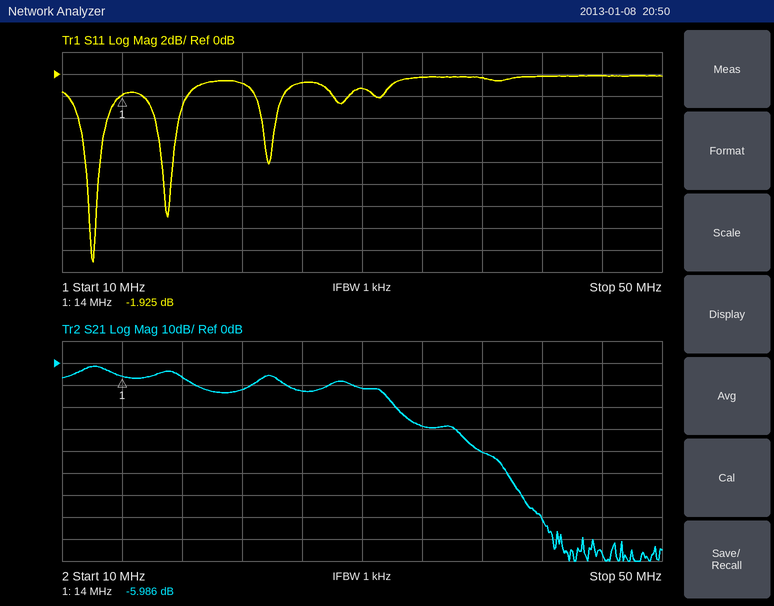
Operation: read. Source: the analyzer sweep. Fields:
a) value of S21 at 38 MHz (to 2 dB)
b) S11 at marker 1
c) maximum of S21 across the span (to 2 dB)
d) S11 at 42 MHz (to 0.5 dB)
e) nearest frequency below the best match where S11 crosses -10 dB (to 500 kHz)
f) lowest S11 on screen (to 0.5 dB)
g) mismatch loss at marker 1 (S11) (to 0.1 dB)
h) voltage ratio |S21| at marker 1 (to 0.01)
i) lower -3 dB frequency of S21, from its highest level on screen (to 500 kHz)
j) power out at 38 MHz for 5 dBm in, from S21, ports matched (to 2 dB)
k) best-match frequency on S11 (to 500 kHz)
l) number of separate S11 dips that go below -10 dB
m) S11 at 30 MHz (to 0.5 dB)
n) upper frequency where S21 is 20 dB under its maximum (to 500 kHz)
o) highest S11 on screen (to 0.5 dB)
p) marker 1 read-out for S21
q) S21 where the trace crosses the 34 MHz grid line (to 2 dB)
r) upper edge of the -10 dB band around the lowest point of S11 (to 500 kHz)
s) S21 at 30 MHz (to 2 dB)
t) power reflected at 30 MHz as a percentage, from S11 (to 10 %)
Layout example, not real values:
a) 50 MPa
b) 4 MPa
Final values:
a) -40 dB
b) -1.925 dB
c) -2 dB
d) 0.0 dB
e) 11.5 MHz
f) -17.0 dB
g) 4.5 dB
h) 0.50
i) 11.0 MHz
j) -36 dBm
k) 12.0 MHz
l) 2
m) -1.5 dB
n) 32.5 MHz
o) 0.0 dB
p) -5.986 dB
q) -28 dB
r) 12.5 MHz
s) -12 dB
t) 70 %
